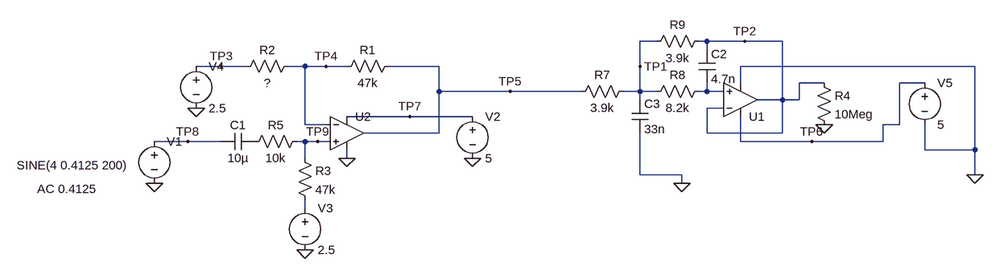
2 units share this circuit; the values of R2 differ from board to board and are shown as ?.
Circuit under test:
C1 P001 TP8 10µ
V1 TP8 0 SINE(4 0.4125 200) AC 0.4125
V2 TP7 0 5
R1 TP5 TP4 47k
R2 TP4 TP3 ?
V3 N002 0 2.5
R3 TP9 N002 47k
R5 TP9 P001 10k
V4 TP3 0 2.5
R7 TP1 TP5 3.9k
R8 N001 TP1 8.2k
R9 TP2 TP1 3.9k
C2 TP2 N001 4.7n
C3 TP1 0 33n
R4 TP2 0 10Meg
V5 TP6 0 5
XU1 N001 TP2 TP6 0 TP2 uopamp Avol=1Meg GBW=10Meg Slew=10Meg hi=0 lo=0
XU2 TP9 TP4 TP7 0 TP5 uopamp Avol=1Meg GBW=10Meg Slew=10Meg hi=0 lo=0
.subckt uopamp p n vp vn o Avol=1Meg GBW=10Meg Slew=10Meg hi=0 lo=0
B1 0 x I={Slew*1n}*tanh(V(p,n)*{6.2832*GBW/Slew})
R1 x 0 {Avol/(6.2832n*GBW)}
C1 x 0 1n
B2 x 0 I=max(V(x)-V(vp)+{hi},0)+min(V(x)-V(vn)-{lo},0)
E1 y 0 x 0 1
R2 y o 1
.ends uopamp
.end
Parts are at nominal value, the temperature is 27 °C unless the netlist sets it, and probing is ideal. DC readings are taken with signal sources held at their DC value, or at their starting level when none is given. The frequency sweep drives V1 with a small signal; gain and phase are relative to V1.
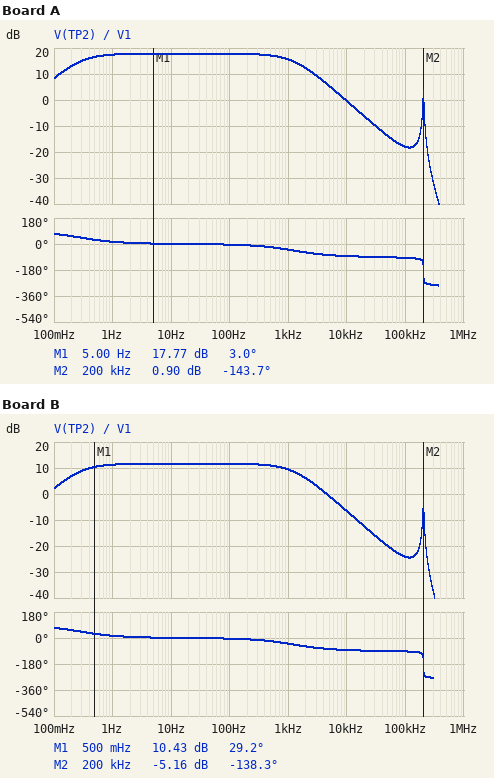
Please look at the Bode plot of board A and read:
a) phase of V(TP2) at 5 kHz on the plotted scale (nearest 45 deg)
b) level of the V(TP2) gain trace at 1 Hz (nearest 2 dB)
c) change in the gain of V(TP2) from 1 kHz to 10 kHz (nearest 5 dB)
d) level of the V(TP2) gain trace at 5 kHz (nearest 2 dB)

-90 deg
18 dB
-15 dB
6 dB
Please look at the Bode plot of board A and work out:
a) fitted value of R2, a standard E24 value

5.6 kΩ
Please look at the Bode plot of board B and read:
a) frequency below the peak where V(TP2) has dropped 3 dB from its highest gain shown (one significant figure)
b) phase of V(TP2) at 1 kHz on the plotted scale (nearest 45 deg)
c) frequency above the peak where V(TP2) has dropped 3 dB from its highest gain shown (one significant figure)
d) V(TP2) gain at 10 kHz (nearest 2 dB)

300 mHz
-45 deg
1 kHz
-6 dB
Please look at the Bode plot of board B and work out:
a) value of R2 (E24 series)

13 kΩ
